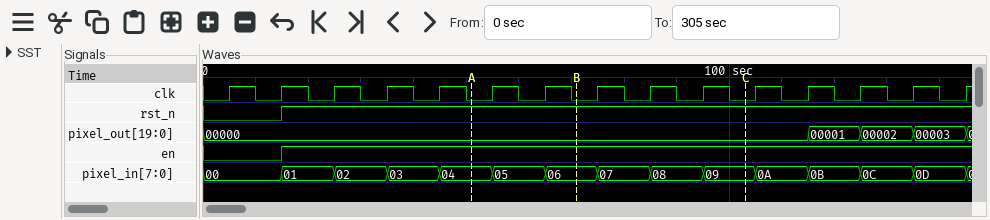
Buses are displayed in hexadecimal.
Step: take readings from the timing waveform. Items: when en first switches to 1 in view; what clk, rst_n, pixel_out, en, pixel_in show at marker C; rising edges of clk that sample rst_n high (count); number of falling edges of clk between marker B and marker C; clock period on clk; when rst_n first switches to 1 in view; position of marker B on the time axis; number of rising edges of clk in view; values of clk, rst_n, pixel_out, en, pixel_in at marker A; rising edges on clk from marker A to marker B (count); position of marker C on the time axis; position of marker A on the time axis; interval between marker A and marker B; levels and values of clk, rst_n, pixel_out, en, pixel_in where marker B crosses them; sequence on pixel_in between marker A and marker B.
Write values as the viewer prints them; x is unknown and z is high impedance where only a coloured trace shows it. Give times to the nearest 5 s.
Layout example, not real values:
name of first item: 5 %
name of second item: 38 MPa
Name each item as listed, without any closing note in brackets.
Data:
when en first switches to 1 in view: 15 s
what clk, rst_n, pixel_out, en, pixel_in show at marker C: clk=0, rst_n=1, pixel_out=00000, en=1, pixel_in=09
rising edges of clk that sample rst_n high: 13
number of falling edges of clk between marker B and marker C: 3
clock period on clk: 10 s
when rst_n first switches to 1 in view: 15 s
position of marker B on the time axis: 70 s
number of rising edges of clk in view: 15
values of clk, rst_n, pixel_out, en, pixel_in at marker A: clk=0, rst_n=1, pixel_out=00000, en=1, pixel_in=04
rising edges on clk from marker A to marker B: 2
position of marker C on the time axis: 105 s
position of marker A on the time axis: 50 s
interval between marker A and marker B: 20 s
levels and values of clk, rst_n, pixel_out, en, pixel_in where marker B crosses them: clk=0, rst_n=1, pixel_out=00000, en=1, pixel_in=06
sequence on pixel_in between marker A and marker B: 04, 05, 06
